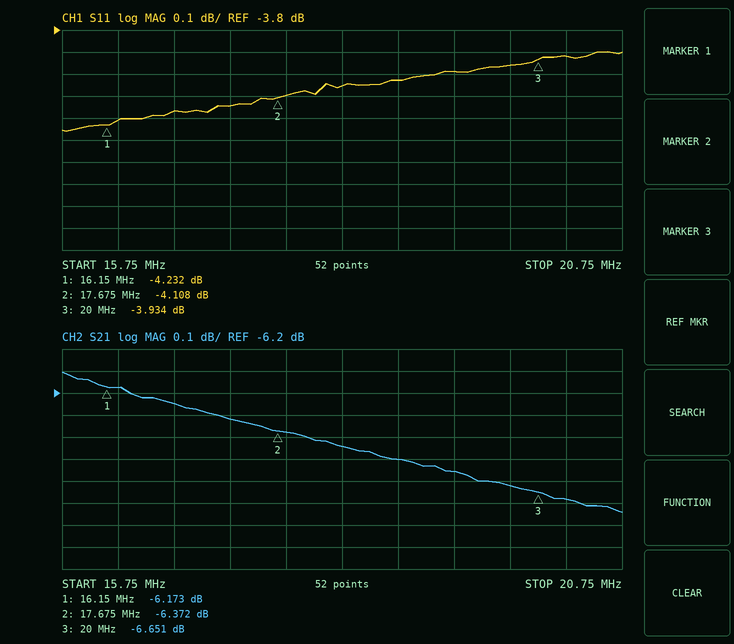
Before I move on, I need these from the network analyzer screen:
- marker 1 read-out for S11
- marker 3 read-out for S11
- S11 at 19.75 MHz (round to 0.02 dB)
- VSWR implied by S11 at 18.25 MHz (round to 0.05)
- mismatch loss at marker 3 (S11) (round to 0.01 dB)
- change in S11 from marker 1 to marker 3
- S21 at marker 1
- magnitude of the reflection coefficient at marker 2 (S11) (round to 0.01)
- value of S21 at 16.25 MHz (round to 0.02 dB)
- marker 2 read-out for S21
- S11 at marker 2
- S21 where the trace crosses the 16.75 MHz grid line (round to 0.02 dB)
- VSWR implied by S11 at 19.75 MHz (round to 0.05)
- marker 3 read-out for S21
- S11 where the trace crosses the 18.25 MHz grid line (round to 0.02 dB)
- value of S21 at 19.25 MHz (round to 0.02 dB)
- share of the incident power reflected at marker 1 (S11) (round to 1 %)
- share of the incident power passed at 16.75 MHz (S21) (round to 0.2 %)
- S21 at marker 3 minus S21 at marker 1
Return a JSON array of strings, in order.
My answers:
["-4.232 dB", "-3.934 dB", "-3.96 dB", "4.35", "2.25 dB", "0.298 dB", "-6.173 dB", "0.62", "-6.18 dB", "-6.372 dB", "-4.108 dB", "-6.24 dB", "4.45", "-6.651 dB", "-4.06 dB", "-6.56 dB", "38 %", "23.8 %", "-0.478 dB"]
